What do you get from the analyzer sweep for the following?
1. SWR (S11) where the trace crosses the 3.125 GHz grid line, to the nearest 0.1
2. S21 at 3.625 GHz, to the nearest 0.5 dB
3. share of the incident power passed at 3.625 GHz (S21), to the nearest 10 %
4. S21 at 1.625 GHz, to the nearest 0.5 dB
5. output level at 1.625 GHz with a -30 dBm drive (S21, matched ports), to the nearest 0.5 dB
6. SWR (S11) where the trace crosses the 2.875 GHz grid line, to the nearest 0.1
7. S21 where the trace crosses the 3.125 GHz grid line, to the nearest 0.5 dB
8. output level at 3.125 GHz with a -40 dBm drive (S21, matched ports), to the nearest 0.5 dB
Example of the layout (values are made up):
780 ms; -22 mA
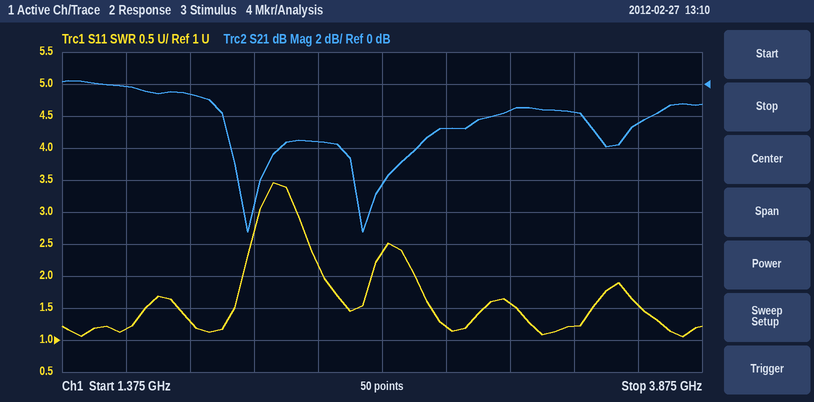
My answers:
1.6; -2.5 dB; 60 %; 0.0 dB; -30.0 dBm; 1.2; -1.5 dB; -41.5 dBm
